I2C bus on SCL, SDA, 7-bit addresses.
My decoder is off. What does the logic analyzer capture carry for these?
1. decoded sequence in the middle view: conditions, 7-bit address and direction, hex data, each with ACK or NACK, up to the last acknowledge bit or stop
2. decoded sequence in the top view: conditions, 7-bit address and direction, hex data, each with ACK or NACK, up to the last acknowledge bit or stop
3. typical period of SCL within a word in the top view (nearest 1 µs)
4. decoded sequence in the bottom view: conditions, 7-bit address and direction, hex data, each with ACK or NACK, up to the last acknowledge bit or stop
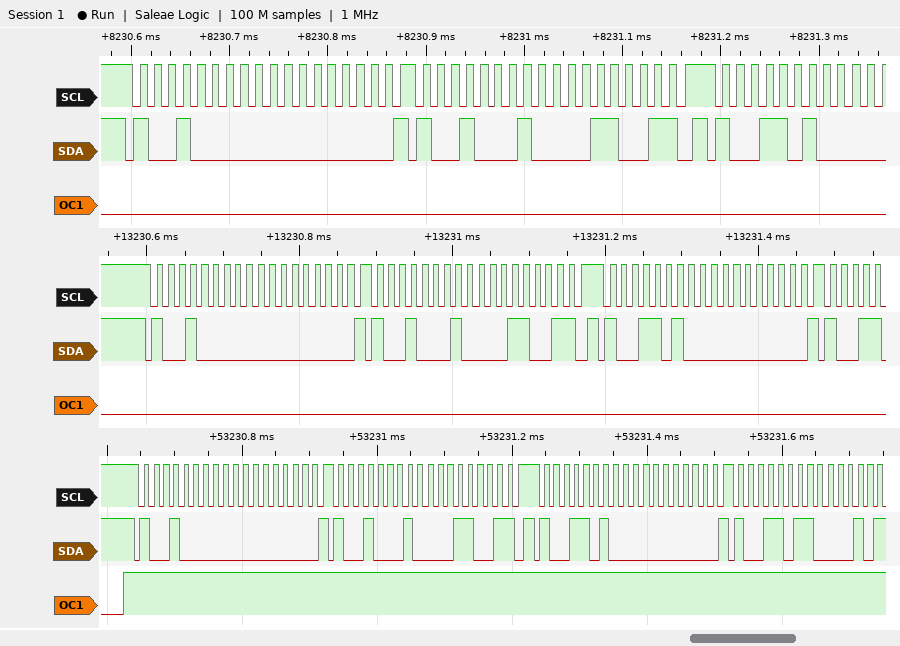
start, address 48 write ACK, 00 ACK, repeated start, address 48 read ACK, 19 NACK, stop, start, address 4D write ACK, 00 ACK
start, address 48 write ACK, 00 ACK, repeated start, address 48 read ACK, 19 NACK, stop, start, address 4D write ACK
15 µs
start, address 48 write ACK, 00 ACK, repeated start, address 48 read ACK, 19 NACK, stop, start, address 4D write ACK, 00 ACK, repeated start, address 4D read ACK
